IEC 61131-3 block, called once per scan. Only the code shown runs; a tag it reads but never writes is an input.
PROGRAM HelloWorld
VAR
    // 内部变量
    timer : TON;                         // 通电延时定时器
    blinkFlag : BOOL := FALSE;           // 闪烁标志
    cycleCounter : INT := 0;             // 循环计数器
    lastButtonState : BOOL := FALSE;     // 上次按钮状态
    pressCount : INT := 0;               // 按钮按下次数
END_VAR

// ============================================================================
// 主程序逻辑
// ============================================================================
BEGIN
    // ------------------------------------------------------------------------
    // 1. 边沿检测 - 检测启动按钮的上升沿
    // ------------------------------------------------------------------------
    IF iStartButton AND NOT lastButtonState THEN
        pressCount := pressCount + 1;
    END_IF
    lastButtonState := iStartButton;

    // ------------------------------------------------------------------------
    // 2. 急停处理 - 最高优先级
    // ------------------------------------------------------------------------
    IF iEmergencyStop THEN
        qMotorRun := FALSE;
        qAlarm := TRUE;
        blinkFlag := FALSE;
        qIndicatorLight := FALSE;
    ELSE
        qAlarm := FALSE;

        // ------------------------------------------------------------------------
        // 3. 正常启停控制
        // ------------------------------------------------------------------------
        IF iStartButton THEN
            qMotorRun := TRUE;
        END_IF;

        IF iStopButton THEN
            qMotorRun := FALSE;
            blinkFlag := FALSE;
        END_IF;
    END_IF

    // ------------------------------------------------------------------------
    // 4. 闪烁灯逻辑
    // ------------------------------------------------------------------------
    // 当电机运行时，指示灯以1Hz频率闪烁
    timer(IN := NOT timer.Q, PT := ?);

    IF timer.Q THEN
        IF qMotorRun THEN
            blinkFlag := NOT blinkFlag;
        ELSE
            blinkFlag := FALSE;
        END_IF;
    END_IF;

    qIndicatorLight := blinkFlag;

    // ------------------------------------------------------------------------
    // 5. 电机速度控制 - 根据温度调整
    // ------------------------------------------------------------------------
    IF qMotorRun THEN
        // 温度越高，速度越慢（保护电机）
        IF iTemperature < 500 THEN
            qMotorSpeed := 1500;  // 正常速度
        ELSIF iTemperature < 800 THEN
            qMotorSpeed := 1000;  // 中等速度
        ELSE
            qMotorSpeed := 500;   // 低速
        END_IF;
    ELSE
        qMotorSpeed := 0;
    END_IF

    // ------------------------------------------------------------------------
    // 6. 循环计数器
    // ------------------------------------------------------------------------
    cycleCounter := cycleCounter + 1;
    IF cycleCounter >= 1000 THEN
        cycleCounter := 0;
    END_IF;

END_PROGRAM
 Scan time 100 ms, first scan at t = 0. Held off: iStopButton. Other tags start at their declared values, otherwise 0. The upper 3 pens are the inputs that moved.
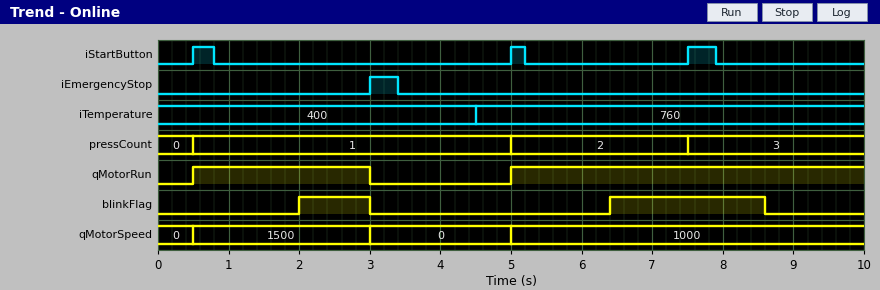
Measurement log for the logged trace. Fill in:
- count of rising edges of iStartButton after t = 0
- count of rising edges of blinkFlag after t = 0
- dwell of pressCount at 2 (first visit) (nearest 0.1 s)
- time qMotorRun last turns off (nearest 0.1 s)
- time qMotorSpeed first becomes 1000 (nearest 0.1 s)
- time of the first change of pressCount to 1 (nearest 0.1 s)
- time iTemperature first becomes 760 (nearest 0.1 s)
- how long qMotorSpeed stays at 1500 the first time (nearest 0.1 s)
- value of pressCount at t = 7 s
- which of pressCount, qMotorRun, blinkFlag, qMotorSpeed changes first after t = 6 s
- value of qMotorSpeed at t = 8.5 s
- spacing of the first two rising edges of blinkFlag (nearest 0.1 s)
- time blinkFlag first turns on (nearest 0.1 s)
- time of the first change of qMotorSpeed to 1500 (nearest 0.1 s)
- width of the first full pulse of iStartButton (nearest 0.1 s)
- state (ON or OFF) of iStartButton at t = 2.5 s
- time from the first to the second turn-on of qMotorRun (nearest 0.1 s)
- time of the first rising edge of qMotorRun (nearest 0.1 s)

3
2
2.5 s
3.0 s
5.0 s
0.5 s
4.5 s
2.5 s
2
blinkFlag
1000
4.4 s
2.0 s
0.5 s
0.3 s
OFF
4.5 s
0.5 s
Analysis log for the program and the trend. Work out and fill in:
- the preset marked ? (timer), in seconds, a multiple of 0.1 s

2.0 s
